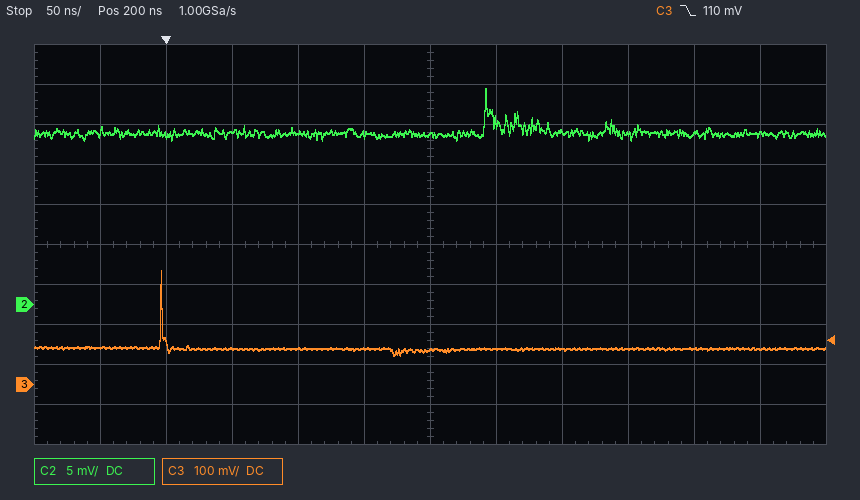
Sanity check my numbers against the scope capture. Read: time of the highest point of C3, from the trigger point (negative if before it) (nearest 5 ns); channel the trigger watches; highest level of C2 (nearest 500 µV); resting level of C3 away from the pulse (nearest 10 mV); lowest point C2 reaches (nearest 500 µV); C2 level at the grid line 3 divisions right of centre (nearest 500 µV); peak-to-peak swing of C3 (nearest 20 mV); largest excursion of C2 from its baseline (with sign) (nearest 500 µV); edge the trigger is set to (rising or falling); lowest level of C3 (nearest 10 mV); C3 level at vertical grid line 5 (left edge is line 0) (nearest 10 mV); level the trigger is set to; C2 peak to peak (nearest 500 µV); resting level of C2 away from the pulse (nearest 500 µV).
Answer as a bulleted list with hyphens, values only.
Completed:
- -5 ns
- C3
- 27.0 mV
- 90 mV
- 20.5 mV
- 21.0 mV
- 220 mV
- +5.5 mV
- falling
- 70 mV
- 90 mV
- 110 mV
- 6.5 mV
- 21.5 mV
